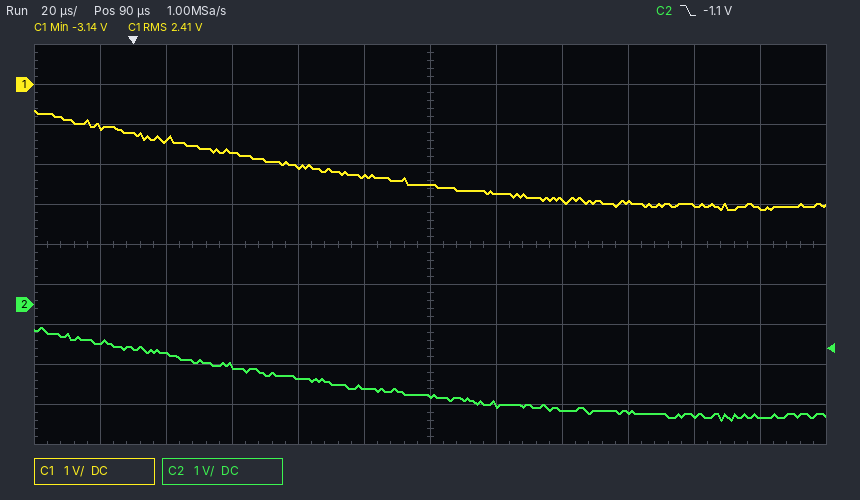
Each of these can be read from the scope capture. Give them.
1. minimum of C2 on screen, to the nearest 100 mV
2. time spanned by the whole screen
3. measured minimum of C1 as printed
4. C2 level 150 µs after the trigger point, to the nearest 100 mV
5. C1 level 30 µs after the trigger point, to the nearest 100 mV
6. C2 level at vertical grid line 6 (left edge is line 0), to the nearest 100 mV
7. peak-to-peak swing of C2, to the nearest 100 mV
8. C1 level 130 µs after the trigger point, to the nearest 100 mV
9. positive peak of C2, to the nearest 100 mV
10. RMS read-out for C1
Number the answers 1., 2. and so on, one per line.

1. -2.9 V
2. 240 µs
3. -3.14 V
4. -2.7 V
5. -1.7 V
6. -2.3 V
7. 2.3 V
8. -2.9 V
9. -600 mV
10. 2.41 V
